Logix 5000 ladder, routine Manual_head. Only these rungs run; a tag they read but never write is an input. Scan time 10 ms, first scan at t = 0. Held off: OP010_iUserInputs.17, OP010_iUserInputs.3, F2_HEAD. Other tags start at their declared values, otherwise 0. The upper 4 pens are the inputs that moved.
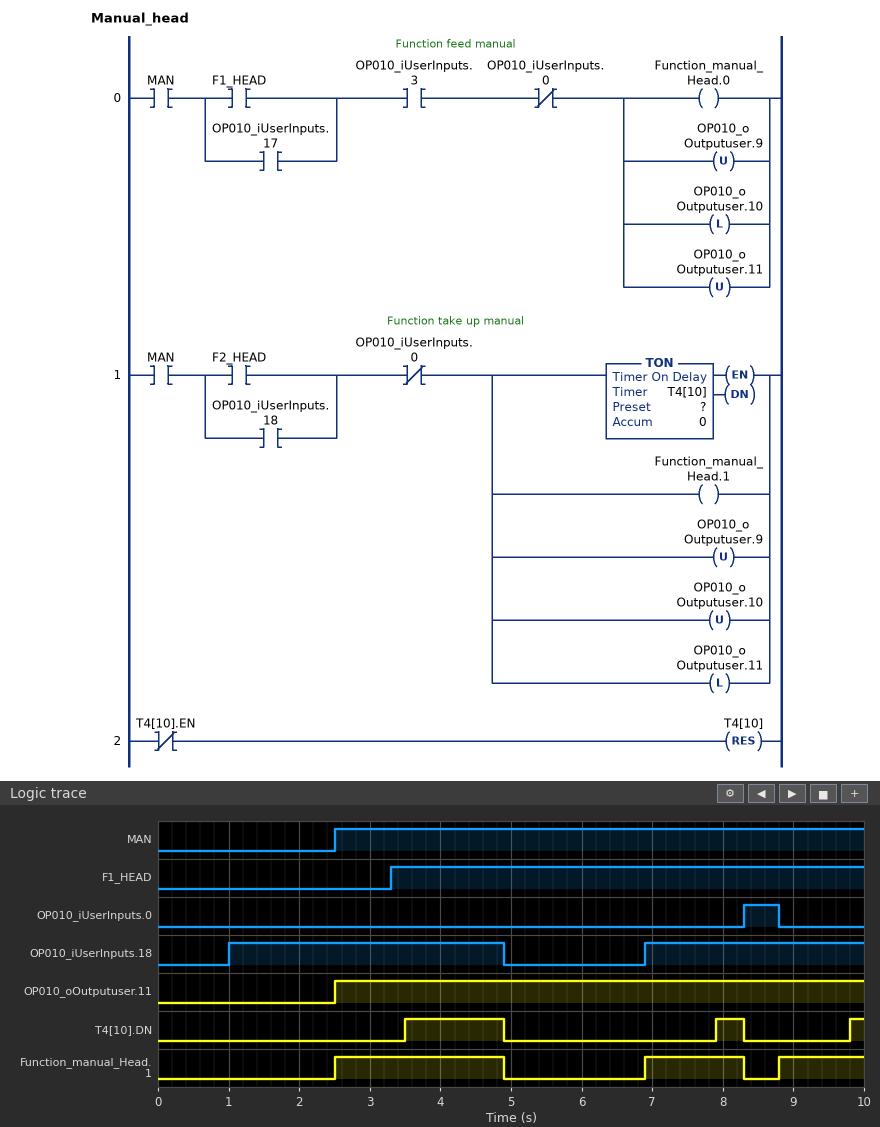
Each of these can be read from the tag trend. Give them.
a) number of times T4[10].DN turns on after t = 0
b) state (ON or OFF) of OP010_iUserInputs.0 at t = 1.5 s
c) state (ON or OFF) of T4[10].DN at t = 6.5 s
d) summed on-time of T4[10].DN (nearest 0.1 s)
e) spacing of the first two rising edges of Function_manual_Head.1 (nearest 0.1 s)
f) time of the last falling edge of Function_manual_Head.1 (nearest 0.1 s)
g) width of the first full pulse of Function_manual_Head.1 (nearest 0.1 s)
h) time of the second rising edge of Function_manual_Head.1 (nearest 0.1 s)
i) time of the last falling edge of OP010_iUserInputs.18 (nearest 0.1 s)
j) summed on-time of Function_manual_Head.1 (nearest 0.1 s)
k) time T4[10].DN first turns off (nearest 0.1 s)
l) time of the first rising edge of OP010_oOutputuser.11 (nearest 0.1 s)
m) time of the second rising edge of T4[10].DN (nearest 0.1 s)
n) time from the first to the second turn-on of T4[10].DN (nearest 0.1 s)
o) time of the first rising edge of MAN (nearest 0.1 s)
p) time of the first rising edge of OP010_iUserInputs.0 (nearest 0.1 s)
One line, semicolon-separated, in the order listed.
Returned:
3; OFF; OFF; 2.0 s; 4.4 s; 8.3 s; 2.4 s; 6.9 s; 4.9 s; 5.0 s; 4.9 s; 2.5 s; 7.9 s; 4.4 s; 2.5 s; 8.3 s
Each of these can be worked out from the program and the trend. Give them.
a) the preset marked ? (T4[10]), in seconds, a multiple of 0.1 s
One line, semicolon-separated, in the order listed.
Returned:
1.0 s
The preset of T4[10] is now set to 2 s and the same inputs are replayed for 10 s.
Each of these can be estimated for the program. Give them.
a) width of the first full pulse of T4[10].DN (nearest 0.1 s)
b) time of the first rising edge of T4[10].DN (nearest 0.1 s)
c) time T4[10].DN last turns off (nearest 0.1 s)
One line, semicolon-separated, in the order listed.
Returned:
0.4 s; 4.5 s; 4.9 s
